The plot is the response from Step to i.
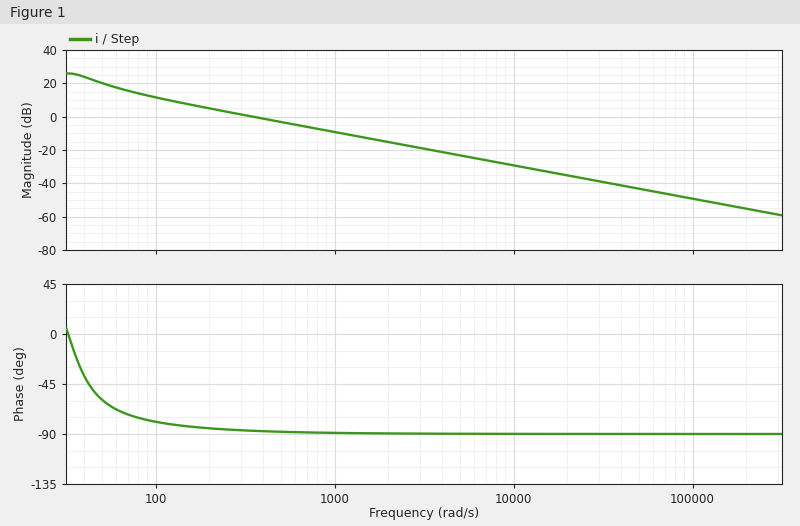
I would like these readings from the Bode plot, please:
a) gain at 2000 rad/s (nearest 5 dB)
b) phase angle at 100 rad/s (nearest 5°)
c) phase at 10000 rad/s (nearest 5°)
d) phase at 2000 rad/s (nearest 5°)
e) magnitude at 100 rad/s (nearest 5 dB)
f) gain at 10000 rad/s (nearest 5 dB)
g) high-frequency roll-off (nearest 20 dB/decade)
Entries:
-15 dB
-80°
-90°
-90°
10 dB
-30 dB
-20 dB/decade
